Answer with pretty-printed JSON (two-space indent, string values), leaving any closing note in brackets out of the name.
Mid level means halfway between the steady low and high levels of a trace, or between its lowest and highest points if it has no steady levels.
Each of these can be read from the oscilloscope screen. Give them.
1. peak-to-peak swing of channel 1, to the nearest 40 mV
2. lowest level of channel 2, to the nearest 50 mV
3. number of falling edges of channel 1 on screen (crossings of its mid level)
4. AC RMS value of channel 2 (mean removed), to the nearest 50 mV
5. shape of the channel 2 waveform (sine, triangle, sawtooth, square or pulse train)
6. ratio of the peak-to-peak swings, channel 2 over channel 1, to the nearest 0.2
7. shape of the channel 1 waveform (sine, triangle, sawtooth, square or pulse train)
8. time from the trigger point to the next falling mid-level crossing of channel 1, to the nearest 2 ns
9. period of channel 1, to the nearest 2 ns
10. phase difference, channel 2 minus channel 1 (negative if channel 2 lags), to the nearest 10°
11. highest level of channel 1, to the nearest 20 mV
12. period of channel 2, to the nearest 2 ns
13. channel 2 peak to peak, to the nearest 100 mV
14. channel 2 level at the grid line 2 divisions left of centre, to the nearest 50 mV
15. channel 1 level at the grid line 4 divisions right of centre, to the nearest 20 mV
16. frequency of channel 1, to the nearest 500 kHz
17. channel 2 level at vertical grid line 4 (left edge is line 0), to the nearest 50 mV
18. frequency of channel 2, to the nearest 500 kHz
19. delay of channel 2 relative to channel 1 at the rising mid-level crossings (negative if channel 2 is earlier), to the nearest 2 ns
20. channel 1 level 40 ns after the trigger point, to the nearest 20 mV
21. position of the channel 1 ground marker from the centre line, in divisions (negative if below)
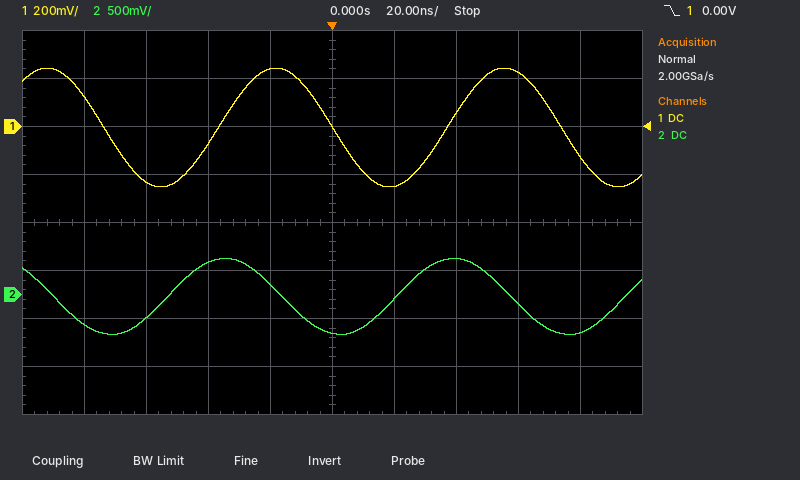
{
  "peak-to-peak swing of channel 1, to the nearest 40 mV": "480 mV",
  "lowest level of channel 2, to the nearest 50 mV": "-400 mV",
  "number of falling edges of channel 1 on screen": "3",
  "AC RMS value of channel 2 (mean removed), to the nearest 50 mV": "300 mV",
  "shape of the channel 2 waveform": "sine",
  "ratio of the peak-to-peak swings, channel 2 over channel 1, to the nearest 0.2": "1.6",
  "shape of the channel 1 waveform": "sine",
  "time from the trigger point to the next falling mid-level crossing of channel 1, to the nearest 2 ns": "74 ns",
  "period of channel 1, to the nearest 2 ns": "74 ns",
  "phase difference, channel 2 minus channel 1 (negative if channel 2 lags), to the nearest 10°": "+80°",
  "highest level of channel 1, to the nearest 20 mV": "240 mV",
  "period of channel 2, to the nearest 2 ns": "74 ns",
  "channel 2 peak to peak, to the nearest 100 mV": "800 mV",
  "channel 2 level at the grid line 2 divisions left of centre, to the nearest 50 mV": "350 mV",
  "channel 1 level at the grid line 4 divisions right of centre, to the nearest 20 mV": "-120 mV",
  "frequency of channel 1, to the nearest 500 kHz": "13.5 MHz",
  "channel 2 level at vertical grid line 4 (left edge is line 0), to the nearest 50 mV": "100 mV",
  "frequency of channel 2, to the nearest 500 kHz": "13.5 MHz",
  "delay of channel 2 relative to channel 1 at the rising mid-level crossings (negative if channel 2 is earlier), to the nearest 2 ns": "-16 ns",
  "channel 1 level 40 ns after the trigger point, to the nearest 20 mV": "60 mV",
  "position of the channel 1 ground marker from the centre line, in divisions": "+2.0 div"
}
